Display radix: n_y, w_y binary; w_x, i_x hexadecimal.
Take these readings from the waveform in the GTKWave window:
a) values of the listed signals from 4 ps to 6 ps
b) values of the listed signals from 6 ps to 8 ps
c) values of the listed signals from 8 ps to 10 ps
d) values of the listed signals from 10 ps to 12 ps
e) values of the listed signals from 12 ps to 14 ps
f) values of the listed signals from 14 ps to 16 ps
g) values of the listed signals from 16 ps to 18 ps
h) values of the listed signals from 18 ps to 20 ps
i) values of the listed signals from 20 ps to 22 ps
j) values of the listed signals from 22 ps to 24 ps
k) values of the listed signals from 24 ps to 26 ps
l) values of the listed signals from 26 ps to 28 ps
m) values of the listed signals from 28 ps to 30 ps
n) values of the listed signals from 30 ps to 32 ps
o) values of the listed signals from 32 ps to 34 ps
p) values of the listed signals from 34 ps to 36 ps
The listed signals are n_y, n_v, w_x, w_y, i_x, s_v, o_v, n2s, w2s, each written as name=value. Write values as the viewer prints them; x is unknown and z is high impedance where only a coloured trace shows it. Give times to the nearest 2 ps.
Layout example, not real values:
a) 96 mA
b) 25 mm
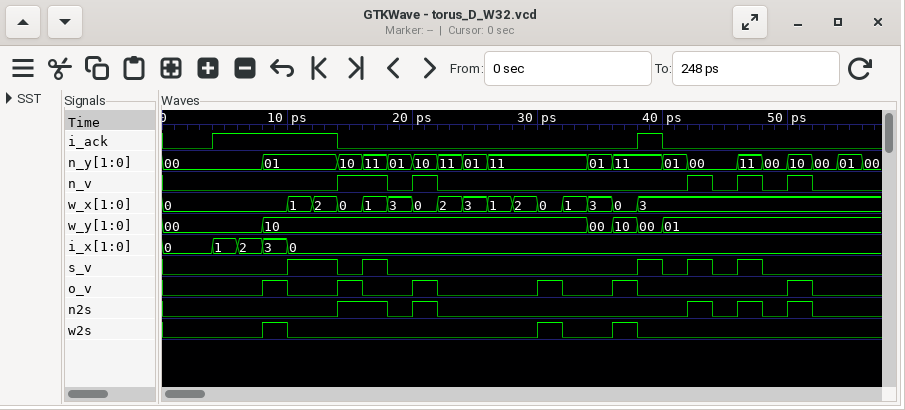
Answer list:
a) n_y=00, n_v=0, w_x=0, w_y=00, i_x=1, s_v=0, o_v=0, n2s=0, w2s=0
b) n_y=00, n_v=0, w_x=0, w_y=00, i_x=2, s_v=0, o_v=0, n2s=0, w2s=0
c) n_y=01, n_v=0, w_x=0, w_y=10, i_x=3, s_v=0, o_v=1, n2s=0, w2s=1
d) n_y=01, n_v=0, w_x=1, w_y=10, i_x=0, s_v=1, o_v=0, n2s=0, w2s=0
e) n_y=01, n_v=0, w_x=2, w_y=10, i_x=0, s_v=1, o_v=0, n2s=0, w2s=0
f) n_y=10, n_v=1, w_x=0, w_y=10, i_x=0, s_v=0, o_v=1, n2s=1, w2s=0
g) n_y=11, n_v=1, w_x=1, w_y=10, i_x=0, s_v=1, o_v=0, n2s=1, w2s=0
h) n_y=01, n_v=0, w_x=3, w_y=10, i_x=0, s_v=0, o_v=0, n2s=0, w2s=0
i) n_y=10, n_v=1, w_x=0, w_y=10, i_x=0, s_v=0, o_v=1, n2s=1, w2s=0
j) n_y=11, n_v=0, w_x=2, w_y=10, i_x=0, s_v=0, o_v=0, n2s=0, w2s=0
k) n_y=01, n_v=0, w_x=3, w_y=10, i_x=0, s_v=0, o_v=0, n2s=0, w2s=0
l) n_y=11, n_v=0, w_x=1, w_y=10, i_x=0, s_v=0, o_v=0, n2s=0, w2s=0
m) n_y=11, n_v=0, w_x=2, w_y=10, i_x=0, s_v=0, o_v=0, n2s=0, w2s=0
n) n_y=11, n_v=0, w_x=0, w_y=10, i_x=0, s_v=0, o_v=1, n2s=0, w2s=1
o) n_y=11, n_v=0, w_x=1, w_y=10, i_x=0, s_v=0, o_v=0, n2s=0, w2s=0
p) n_y=01, n_v=0, w_x=3, w_y=00, i_x=0, s_v=0, o_v=0, n2s=0, w2s=0
